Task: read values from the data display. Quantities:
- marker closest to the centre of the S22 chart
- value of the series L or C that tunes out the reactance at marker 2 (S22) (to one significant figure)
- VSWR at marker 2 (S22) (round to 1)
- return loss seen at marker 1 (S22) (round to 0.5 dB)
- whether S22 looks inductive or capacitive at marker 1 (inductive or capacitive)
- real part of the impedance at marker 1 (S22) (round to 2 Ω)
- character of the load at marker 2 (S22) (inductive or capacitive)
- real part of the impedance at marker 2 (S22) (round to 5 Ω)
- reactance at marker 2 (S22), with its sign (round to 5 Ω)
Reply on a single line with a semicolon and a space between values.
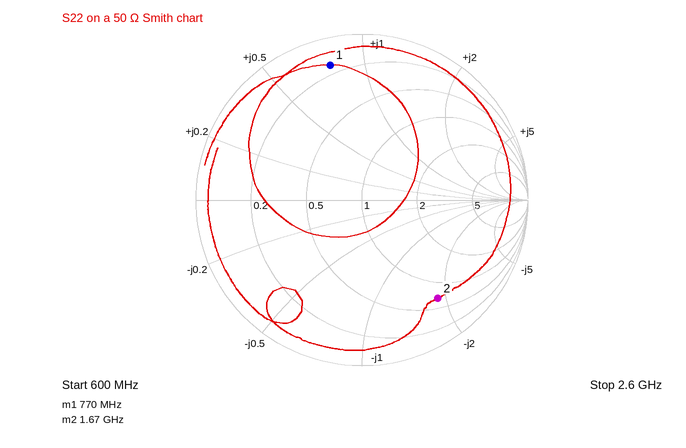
marker 2; 9 nH; 7; 1.5 dB; inductive; 8 Ω; capacitive; 35 Ω; -90 Ω
